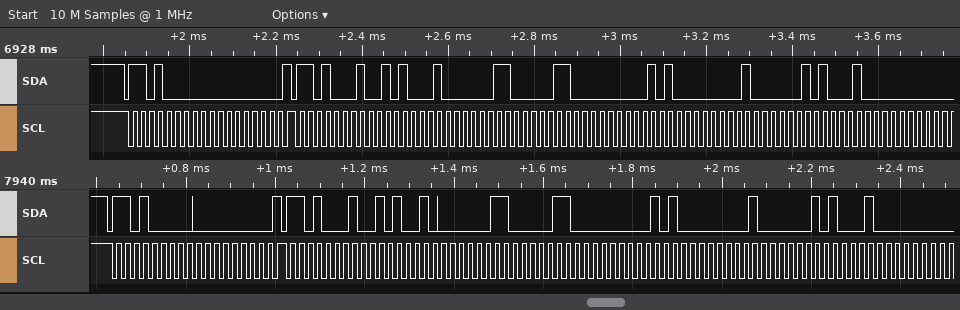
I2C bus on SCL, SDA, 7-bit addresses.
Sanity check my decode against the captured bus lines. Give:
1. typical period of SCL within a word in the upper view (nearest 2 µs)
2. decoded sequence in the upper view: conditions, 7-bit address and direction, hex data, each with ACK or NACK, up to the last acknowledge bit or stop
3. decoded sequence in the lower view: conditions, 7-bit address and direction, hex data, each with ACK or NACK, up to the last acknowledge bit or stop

20 µs
start, address 68 write ACK, 00 ACK, repeated start, address 68 read ACK, 51 ACK, 06 ACK, 18 ACK, 05 ACK, 01 ACK, 05 ACK, 20 ACK
start, address 68 write ACK, 00 ACK, repeated start, address 68 read ACK, 52 ACK, 06 ACK, 18 ACK, 05 ACK, 01 ACK, 05 ACK, 20 ACK
